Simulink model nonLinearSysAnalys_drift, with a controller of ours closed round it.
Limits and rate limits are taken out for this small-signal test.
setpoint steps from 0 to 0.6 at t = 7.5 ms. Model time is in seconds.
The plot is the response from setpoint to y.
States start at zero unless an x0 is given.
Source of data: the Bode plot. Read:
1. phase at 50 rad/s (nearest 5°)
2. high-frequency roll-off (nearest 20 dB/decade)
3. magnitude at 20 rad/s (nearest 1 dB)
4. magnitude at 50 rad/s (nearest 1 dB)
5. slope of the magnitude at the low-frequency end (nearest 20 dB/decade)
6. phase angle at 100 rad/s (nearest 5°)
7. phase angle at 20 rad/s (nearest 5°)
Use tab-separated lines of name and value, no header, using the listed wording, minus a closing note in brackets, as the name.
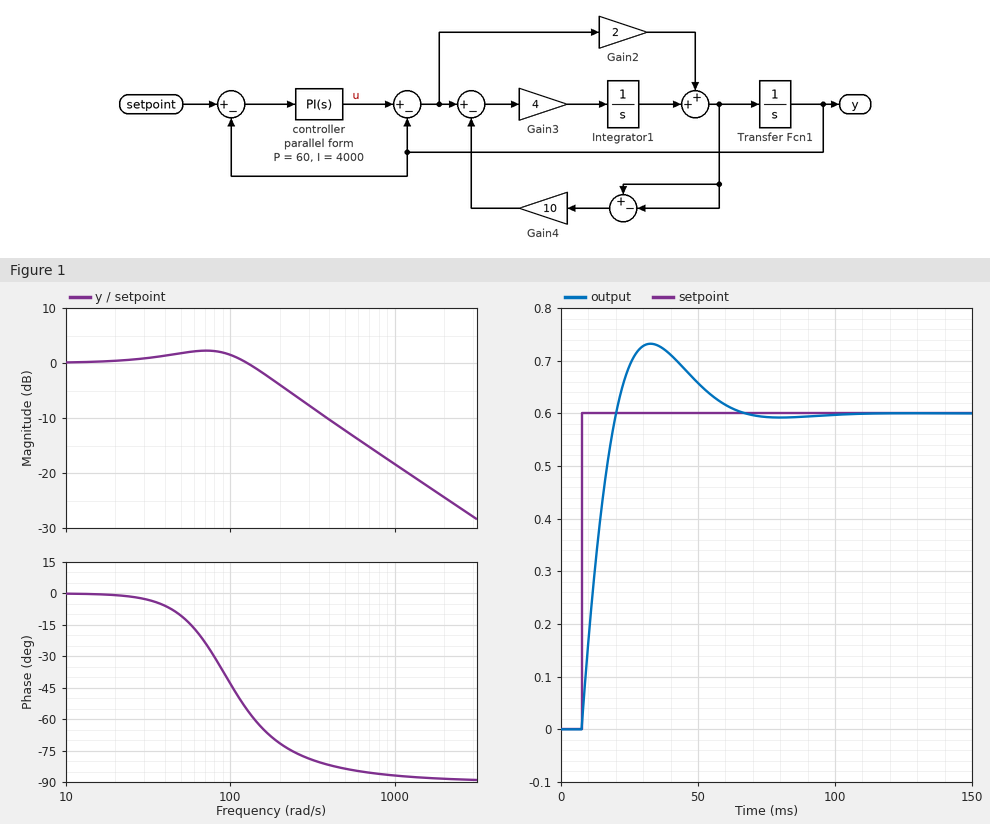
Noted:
phase at 50 rad/s	-10°
high-frequency roll-off	-20 dB/decade
magnitude at 20 rad/s	0 dB
magnitude at 50 rad/s	2 dB
slope of the magnitude at the low-frequency end	0 dB/decade
phase angle at 100 rad/s	-45°
phase angle at 20 rad/s	0°
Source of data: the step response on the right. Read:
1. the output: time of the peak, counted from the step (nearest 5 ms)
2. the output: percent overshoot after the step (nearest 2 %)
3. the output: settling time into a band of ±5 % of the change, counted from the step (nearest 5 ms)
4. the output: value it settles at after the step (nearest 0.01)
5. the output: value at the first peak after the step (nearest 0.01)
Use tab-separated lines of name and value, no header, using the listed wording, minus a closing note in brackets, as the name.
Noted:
the output: time of the peak, counted from the step	25 ms
the output: percent overshoot after the step	22 %
the output: settling time into a band of ±5 % of the change, counted from the step	50 ms
the output: value it settles at after the step	0.60
the output: value at the first peak after the step	0.73
